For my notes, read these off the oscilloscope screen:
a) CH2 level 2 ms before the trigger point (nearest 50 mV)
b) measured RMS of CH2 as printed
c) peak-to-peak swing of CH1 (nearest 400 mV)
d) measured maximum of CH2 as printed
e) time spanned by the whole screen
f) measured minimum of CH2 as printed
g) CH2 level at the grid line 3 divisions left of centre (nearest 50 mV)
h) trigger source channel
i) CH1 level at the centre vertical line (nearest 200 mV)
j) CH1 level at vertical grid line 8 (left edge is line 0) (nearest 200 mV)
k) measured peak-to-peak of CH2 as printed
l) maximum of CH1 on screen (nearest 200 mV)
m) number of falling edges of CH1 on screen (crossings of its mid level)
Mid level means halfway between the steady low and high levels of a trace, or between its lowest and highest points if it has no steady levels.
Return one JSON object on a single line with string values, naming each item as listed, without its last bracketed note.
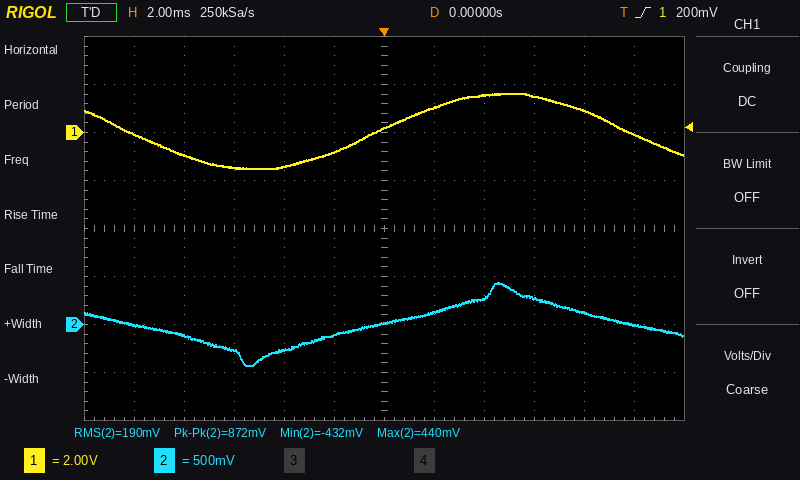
{"CH2 level 2 ms before the trigger point": "-100 mV", "measured RMS of CH2 as printed": "190 mV", "peak-to-peak swing of CH1": "3.2 V", "measured maximum of CH2 as printed": "440 mV", "time spanned by the whole screen": "24 ms", "measured minimum of CH2 as printed": "-432 mV", "CH2 level at the grid line 3 divisions left of centre": "-250 mV", "trigger source channel": "CH1", "CH1 level at the centre vertical line": "200 mV", "CH1 level at vertical grid line 8 (left edge is line 0)": "1.6 V", "measured peak-to-peak of CH2 as printed": "872 mV", "maximum of CH1 on screen": "1.6 V", "number of falling edges of CH1 on screen": "2"}
